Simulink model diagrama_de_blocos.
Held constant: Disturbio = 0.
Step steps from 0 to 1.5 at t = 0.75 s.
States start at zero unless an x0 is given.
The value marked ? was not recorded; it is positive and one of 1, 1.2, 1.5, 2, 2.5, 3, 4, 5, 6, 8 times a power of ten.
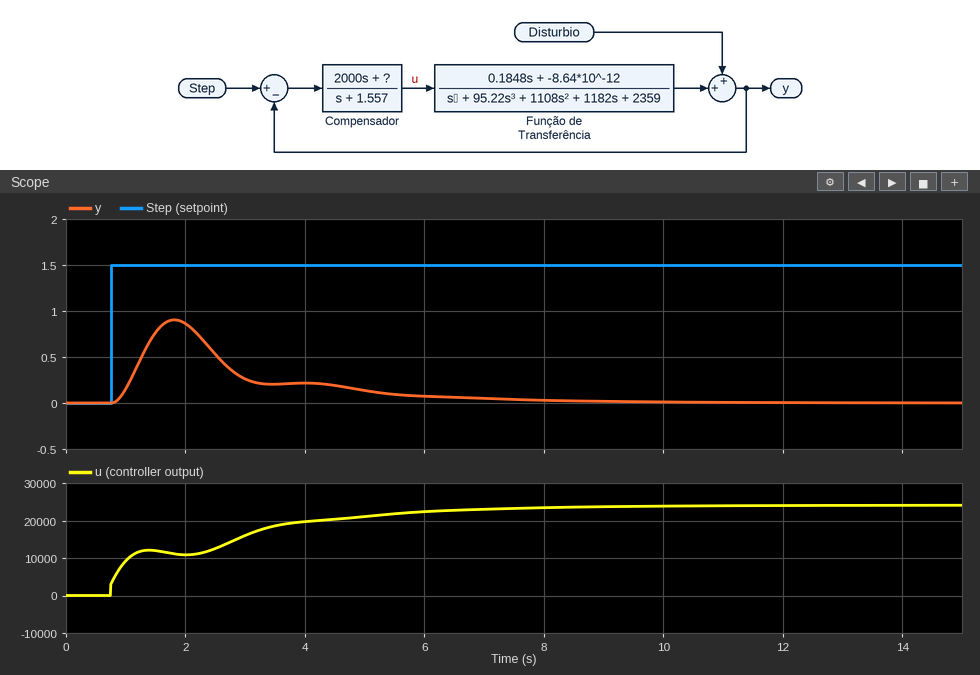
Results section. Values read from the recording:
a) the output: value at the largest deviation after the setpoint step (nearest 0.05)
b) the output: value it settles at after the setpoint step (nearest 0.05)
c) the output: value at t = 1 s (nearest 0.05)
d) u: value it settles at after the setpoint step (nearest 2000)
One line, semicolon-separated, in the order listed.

0.90; 0.00; 0.15; 24000
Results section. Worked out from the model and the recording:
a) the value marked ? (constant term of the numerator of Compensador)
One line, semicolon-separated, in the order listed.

25000
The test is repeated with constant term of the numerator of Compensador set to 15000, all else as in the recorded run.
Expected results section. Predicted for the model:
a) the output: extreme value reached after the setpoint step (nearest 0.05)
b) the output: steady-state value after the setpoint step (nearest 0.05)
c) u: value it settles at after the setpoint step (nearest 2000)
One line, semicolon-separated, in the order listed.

0.65; 0.00; 14000
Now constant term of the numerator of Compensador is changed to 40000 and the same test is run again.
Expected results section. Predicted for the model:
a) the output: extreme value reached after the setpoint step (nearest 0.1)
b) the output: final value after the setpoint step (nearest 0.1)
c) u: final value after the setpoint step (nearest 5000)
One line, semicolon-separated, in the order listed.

1.2; 0.0; 40000
